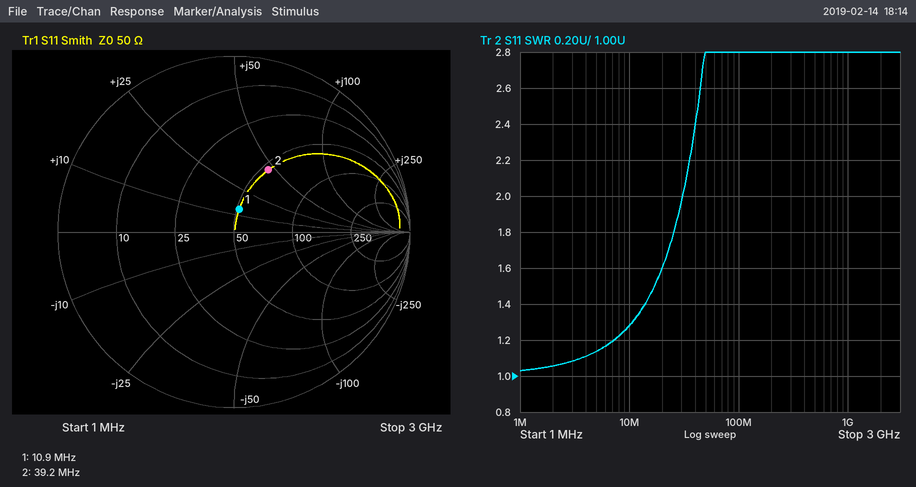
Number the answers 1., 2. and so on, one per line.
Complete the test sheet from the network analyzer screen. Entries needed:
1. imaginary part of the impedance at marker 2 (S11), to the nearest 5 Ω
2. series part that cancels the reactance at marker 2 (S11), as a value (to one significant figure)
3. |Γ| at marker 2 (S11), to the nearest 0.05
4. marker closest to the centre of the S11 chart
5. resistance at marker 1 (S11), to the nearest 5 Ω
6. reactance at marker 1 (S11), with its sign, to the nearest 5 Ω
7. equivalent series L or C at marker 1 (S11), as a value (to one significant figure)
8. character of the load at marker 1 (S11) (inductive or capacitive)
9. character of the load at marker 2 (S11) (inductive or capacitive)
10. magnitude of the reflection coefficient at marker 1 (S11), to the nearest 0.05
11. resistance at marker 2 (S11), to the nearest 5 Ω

1. +45 Ω
2. 90 pF
3. 0.40
4. marker 1
5. 50 Ω
6. +15 Ω
7. 200 nH
8. inductive
9. inductive
10. 0.15
11. 55 Ω
